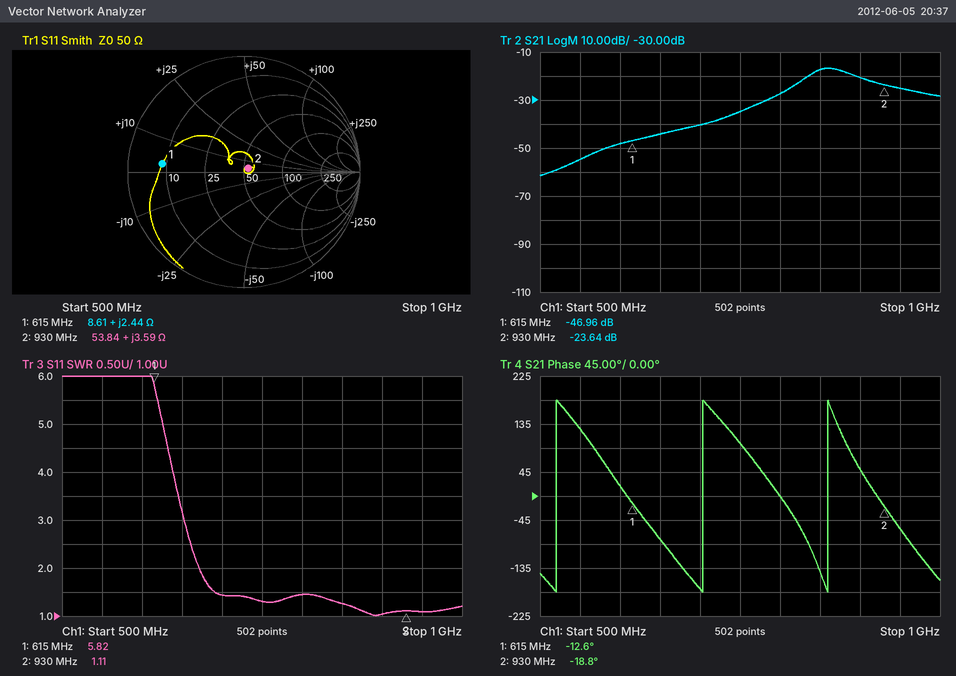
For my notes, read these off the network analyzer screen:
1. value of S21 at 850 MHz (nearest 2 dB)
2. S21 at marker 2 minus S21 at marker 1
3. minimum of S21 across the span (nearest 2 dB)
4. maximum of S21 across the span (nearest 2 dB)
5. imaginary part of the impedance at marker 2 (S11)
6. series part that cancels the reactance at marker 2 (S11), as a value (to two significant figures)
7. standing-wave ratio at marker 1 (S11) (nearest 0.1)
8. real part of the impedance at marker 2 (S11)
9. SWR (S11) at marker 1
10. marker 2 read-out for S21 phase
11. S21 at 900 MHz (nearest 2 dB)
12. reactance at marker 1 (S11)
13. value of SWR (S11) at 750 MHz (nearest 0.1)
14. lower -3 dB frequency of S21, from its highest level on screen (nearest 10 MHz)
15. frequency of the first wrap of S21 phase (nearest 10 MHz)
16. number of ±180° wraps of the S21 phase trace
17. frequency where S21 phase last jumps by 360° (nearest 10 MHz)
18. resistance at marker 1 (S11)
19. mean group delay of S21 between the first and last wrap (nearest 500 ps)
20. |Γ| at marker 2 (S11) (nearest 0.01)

-18 dB
23.32 dB
-62 dB
-16 dB
+3.59 Ω
48 pF
5.8
53.84 Ω
5.82
-18.8°
-20 dB
+2.44 Ω
1.3
840 MHz
520 MHz
3
860 MHz
8.61 Ω
6.0 ns
0.05
